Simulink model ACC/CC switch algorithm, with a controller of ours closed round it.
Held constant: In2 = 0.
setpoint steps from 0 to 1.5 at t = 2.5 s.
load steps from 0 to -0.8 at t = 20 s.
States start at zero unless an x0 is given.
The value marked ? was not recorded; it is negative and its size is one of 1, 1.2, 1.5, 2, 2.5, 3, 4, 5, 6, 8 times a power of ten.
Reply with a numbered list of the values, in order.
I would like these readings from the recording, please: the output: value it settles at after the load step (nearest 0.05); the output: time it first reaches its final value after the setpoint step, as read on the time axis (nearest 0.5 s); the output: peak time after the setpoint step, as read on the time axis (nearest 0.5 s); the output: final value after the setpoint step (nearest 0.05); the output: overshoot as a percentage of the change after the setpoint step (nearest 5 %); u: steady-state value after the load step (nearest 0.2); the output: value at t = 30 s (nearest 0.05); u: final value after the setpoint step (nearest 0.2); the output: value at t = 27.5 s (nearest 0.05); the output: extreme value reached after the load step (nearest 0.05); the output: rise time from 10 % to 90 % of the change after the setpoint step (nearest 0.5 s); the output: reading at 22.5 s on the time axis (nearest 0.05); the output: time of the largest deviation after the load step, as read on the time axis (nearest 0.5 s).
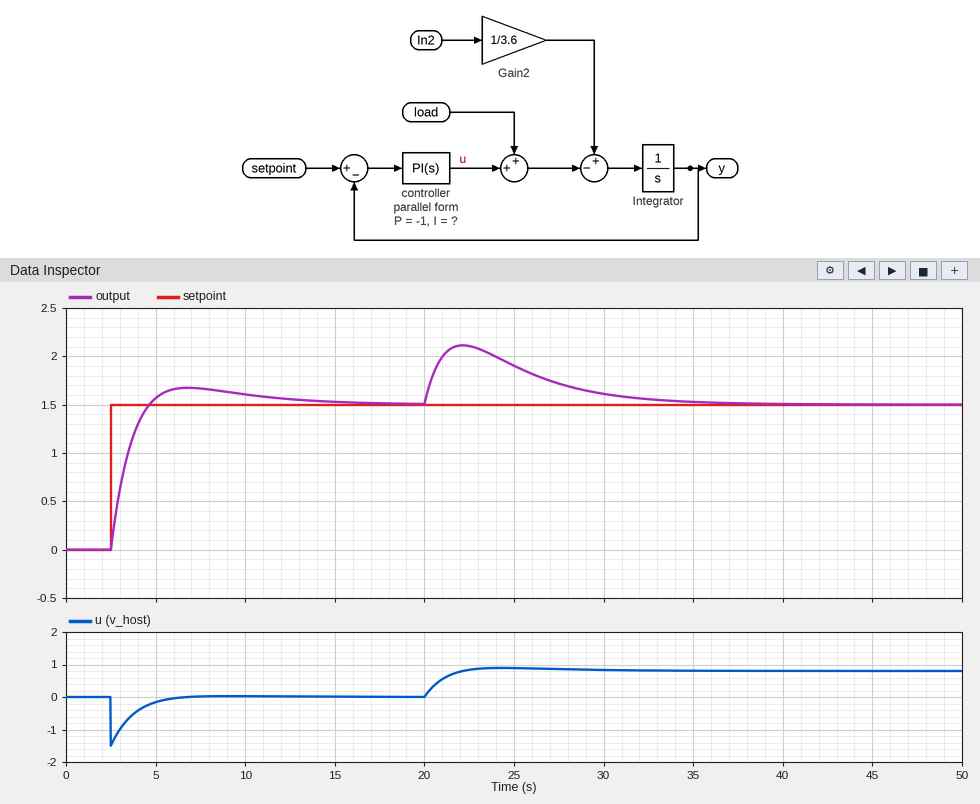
1. 1.50
2. 4.5 s
3. 7.0 s
4. 1.50
5. 10 %
6. 0.8
7. 1.60
8. 0.0
9. 1.70
10. 2.10
11. 1.5 s
12. 2.10
13. 22.0 s
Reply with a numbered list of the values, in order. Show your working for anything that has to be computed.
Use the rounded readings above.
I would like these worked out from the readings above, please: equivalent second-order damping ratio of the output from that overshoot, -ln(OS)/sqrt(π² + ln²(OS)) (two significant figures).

1. ln(0.1) = -2.303; 2.303 / sqrt(9.870 + 5.302) = 0.59
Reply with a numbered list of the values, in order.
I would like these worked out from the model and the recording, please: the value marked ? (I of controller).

1. -0.2
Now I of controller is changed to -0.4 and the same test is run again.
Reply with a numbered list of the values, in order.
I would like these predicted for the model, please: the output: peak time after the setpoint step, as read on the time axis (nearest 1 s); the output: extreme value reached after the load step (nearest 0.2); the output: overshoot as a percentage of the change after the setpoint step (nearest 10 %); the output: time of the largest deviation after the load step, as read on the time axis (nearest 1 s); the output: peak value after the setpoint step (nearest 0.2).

1. 6 s
2. 2.0
3. 20 %
4. 22 s
5. 1.8
